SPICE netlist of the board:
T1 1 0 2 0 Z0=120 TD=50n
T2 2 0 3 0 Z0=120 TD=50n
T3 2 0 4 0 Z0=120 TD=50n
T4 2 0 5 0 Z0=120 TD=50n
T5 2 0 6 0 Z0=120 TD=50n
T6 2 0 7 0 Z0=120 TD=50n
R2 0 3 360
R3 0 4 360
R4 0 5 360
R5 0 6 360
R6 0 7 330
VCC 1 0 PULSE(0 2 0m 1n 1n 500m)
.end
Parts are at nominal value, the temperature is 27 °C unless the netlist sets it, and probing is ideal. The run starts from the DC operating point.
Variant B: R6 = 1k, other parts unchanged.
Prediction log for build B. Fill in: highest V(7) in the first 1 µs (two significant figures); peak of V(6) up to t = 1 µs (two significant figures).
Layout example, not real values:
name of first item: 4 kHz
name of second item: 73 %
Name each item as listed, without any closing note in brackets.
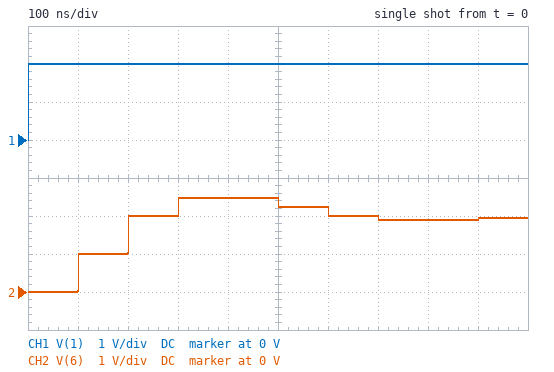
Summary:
highest V(7) in the first 1 µs: 2.7 V
peak of V(6) up to t = 1 µs: 2.6 V
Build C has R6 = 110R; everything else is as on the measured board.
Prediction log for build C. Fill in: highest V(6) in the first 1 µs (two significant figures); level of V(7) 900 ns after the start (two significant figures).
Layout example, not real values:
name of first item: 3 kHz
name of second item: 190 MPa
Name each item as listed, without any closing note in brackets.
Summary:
highest V(6) in the first 1 µs: 2.2 V
level of V(7) 900 ns after the start: 2.0 V
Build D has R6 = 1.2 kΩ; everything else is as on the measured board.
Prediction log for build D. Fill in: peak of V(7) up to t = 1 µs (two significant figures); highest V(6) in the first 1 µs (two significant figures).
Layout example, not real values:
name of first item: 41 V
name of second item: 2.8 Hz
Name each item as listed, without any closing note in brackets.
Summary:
peak of V(7) up to t = 1 µs: 2.7 V
highest V(6) in the first 1 µs: 2.6 V
